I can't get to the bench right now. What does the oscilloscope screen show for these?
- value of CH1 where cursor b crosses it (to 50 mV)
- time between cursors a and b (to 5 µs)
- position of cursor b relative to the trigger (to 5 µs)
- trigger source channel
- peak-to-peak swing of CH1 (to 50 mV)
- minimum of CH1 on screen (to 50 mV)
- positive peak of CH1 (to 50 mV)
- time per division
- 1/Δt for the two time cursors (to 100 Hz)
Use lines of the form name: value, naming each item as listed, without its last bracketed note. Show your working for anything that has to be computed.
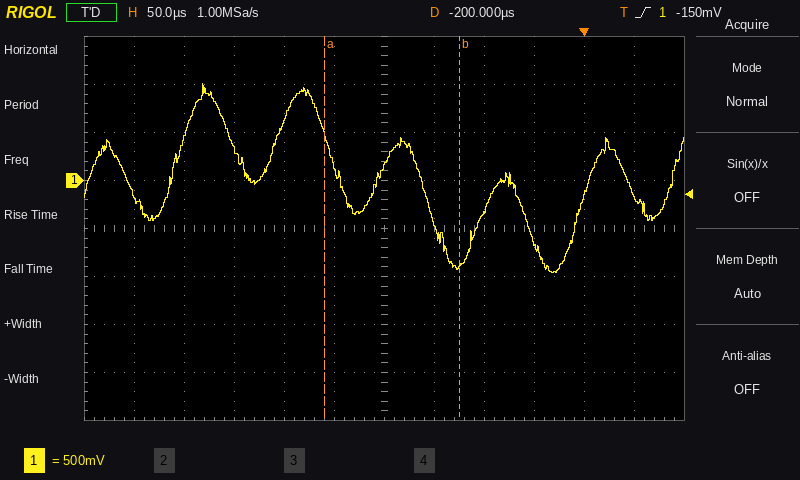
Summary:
value of CH1 where cursor b crosses it: -900 mV
time between cursors a and b: 135 µs
position of cursor b relative to the trigger: -125 µs
trigger source channel: CH1
peak-to-peak swing of CH1: 1.00 V − (-950 mV) = 1.95 V
minimum of CH1 on screen: -950 mV
positive peak of CH1: 1.00 V
time per division: 50 µs
1/Δt for the two time cursors: 1 / 135 µs ≈ 7.4 kHz
